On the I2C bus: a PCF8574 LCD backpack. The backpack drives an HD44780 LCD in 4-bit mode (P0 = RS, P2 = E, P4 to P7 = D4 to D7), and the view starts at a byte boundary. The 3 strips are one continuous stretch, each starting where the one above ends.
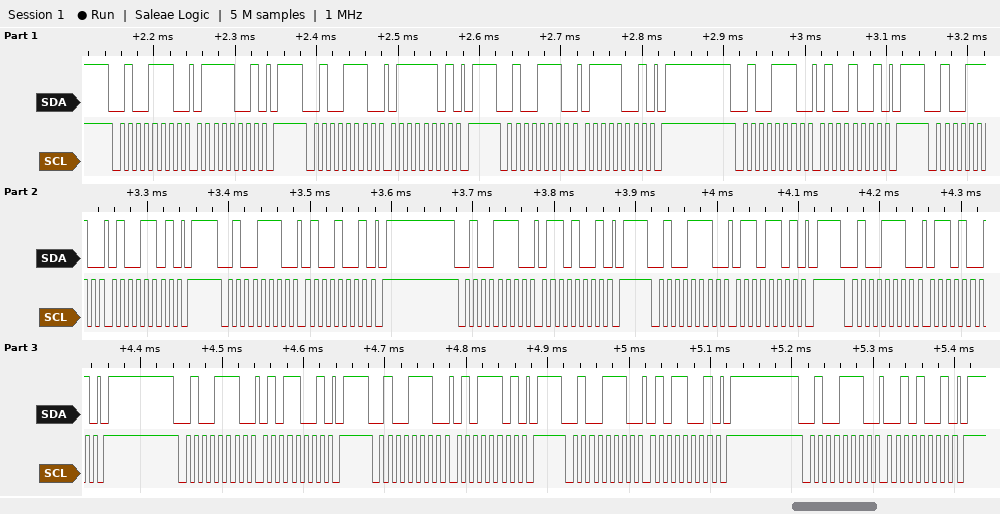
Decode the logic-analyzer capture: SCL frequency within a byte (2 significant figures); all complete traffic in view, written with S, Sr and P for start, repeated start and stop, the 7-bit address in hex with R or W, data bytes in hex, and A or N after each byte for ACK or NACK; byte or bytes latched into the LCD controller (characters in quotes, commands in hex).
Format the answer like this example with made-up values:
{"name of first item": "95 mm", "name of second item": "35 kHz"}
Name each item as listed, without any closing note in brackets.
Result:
{"SCL frequency within a byte": "100 kHz", "all complete traffic in view, written with S, Sr and P for start, repeated start and stop, the 7-bit address in hex with R or W, data bytes in hex, and A or N after each byte for ACK or NACK": "S 27W A 79 A P S 27W A 7D A P S 27W A 79 A P S 27W A 49 A P S 27W A 4D A P S 27W A 49 A P S 27W A 69 A P S 27W A 6D A P S 27W A 69 A P S 27W A 59 A P S 27W A 5D A P S 27W A 59 A P S 27W A 29 A P", "byte or bytes latched into the LCD controller": "'t' 'e'"}
